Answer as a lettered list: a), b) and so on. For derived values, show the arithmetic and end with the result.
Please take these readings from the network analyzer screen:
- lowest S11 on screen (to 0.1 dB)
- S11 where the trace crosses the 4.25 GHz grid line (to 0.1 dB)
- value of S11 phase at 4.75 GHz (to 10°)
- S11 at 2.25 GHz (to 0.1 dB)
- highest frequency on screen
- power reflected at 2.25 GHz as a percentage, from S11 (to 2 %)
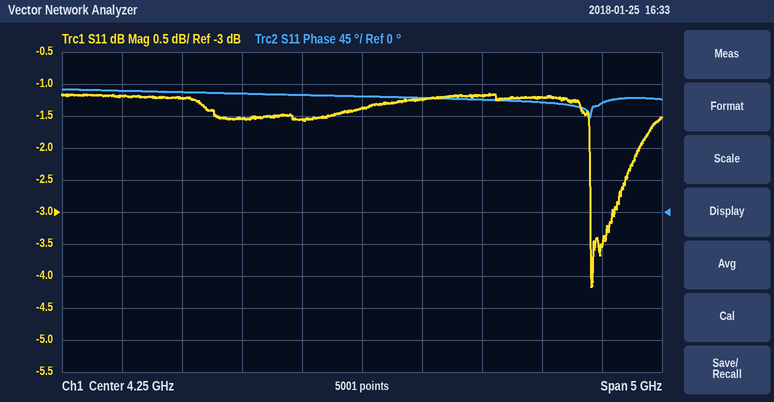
a) -4.2 dB
b) -1.4 dB
c) 160°
d) -1.2 dB
e) 6.75 GHz
f) 10^(-1.2/10) ≈ 76 %
